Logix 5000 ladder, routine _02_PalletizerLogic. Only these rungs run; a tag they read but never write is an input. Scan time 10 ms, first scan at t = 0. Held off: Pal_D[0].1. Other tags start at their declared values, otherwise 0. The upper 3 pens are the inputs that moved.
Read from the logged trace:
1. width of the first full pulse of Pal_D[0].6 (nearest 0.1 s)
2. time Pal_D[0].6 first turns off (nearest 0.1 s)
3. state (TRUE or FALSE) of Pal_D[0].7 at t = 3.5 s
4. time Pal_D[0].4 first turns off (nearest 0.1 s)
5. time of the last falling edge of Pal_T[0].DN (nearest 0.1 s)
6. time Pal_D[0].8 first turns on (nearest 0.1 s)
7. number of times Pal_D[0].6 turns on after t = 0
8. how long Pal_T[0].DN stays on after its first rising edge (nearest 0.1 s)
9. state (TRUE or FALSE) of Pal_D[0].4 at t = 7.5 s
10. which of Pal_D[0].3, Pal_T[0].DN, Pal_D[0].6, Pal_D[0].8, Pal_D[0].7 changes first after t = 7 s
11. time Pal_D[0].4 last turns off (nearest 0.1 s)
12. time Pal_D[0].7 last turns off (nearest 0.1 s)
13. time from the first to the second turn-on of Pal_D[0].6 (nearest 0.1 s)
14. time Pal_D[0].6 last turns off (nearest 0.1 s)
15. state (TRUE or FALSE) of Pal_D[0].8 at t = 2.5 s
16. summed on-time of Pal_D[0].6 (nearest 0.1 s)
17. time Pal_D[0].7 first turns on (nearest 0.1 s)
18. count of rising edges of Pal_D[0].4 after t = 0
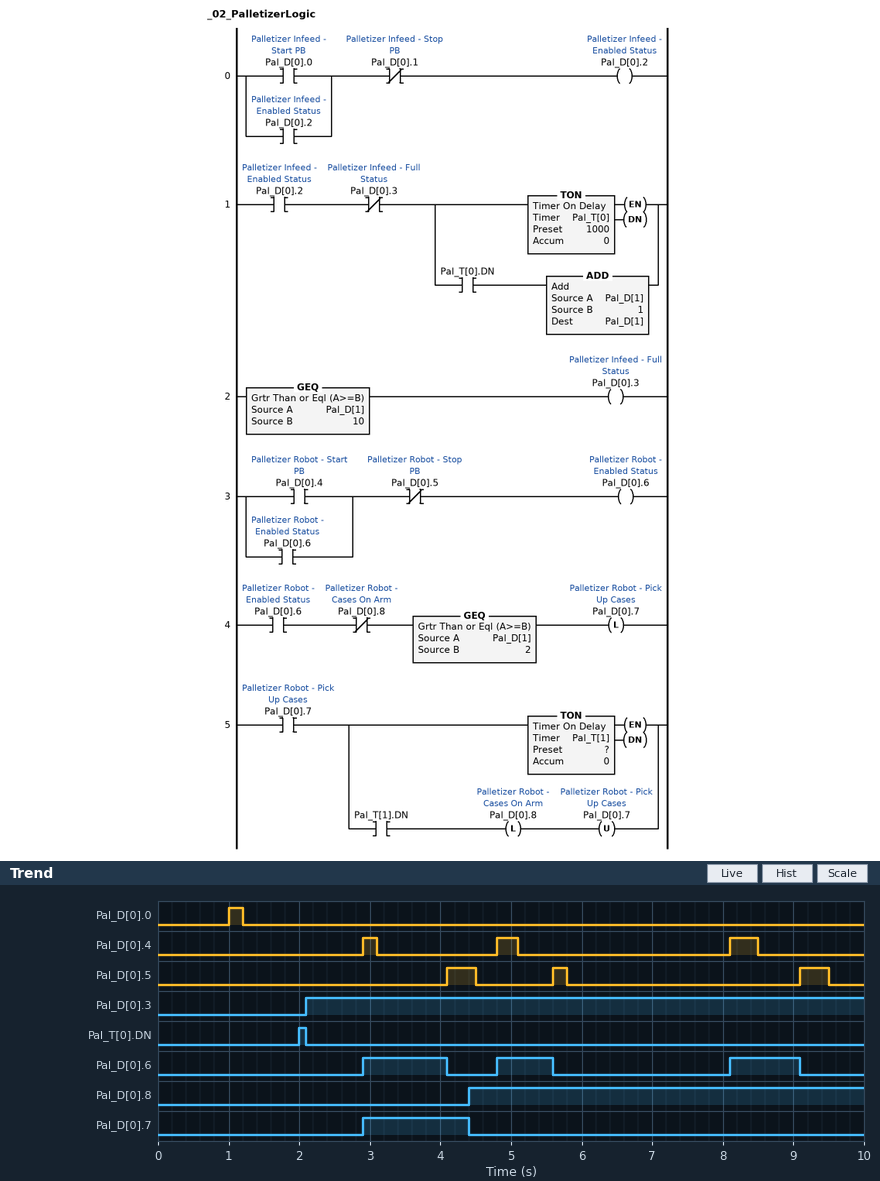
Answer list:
1.2 s
4.1 s
TRUE
3.1 s
2.1 s
4.4 s
3
0.1 s
FALSE
Pal_D[0].6
8.5 s
4.4 s
1.9 s
9.1 s
FALSE
3.0 s
2.9 s
3
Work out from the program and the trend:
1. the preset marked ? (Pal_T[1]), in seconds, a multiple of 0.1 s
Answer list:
1.5 s
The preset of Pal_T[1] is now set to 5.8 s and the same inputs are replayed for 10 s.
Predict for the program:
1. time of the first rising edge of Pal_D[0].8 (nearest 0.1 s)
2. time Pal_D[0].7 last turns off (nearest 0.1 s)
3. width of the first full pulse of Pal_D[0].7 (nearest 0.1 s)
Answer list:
8.7 s
8.7 s
5.8 s
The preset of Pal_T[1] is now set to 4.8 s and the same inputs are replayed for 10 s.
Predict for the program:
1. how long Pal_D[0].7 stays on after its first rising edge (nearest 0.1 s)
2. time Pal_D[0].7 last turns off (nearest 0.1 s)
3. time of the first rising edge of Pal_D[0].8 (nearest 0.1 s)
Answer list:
4.8 s
7.7 s
7.7 s
